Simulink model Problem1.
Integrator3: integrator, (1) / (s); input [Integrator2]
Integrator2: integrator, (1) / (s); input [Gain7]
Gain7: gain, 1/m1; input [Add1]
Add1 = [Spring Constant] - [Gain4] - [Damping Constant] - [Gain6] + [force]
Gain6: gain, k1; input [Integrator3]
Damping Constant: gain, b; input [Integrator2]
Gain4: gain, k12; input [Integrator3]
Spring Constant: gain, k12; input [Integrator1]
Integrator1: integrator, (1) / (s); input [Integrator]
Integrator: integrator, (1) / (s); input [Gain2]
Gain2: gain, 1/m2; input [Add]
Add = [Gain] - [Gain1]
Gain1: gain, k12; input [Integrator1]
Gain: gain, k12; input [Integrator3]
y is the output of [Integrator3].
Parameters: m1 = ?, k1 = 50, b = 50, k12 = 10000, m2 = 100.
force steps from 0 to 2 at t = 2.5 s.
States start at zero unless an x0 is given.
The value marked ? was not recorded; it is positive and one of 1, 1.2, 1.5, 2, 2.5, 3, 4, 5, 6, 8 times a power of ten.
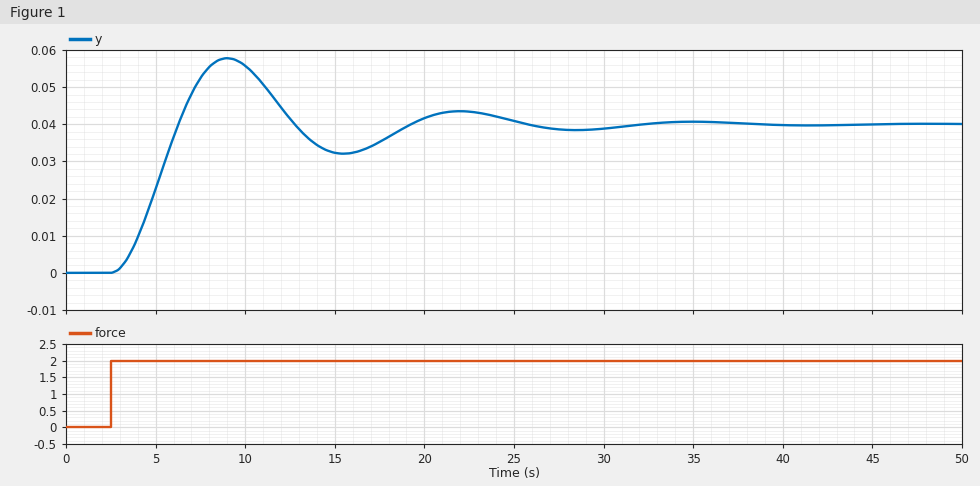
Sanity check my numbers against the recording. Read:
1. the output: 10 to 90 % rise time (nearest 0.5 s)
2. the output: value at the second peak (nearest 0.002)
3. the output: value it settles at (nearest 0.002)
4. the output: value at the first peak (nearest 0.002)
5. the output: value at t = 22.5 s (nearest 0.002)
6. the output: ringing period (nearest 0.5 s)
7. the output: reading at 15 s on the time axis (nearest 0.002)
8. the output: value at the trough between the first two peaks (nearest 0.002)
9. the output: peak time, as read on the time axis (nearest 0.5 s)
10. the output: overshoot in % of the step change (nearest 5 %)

2.5 s
0.044
0.040
0.058
0.044
13.0 s
0.032
0.032
9.0 s
45 %
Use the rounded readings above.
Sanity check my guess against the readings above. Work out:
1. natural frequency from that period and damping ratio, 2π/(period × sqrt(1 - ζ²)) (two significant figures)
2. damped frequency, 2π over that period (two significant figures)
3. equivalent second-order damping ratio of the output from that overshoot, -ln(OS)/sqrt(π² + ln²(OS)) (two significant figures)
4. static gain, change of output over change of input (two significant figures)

0.50 rad/s
0.48 rad/s
0.25
0.020
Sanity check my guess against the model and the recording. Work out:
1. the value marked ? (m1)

100
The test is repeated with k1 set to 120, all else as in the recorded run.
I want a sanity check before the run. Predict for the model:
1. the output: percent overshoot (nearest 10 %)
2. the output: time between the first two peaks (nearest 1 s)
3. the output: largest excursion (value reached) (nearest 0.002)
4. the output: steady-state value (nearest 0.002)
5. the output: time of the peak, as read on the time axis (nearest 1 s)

60 %
8 s
0.026
0.016
7 s
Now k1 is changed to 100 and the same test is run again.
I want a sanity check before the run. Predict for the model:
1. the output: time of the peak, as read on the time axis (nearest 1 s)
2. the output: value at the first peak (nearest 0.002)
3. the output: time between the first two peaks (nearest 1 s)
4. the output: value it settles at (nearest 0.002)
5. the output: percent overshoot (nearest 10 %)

7 s
0.032
9 s
0.020
60 %
